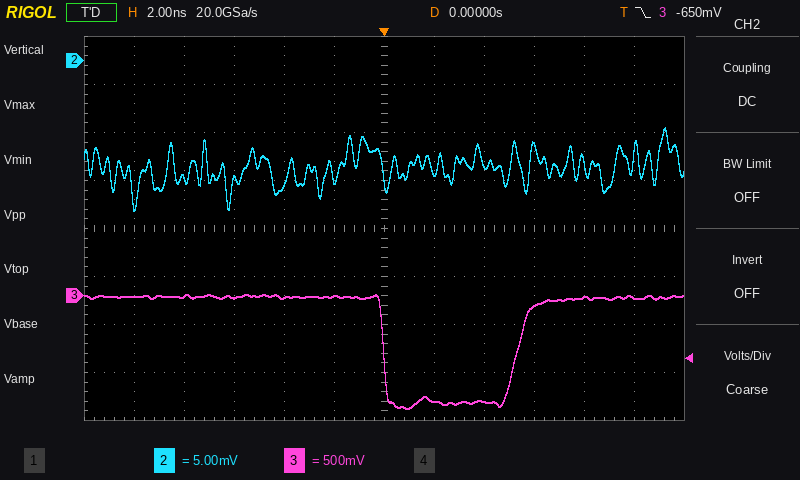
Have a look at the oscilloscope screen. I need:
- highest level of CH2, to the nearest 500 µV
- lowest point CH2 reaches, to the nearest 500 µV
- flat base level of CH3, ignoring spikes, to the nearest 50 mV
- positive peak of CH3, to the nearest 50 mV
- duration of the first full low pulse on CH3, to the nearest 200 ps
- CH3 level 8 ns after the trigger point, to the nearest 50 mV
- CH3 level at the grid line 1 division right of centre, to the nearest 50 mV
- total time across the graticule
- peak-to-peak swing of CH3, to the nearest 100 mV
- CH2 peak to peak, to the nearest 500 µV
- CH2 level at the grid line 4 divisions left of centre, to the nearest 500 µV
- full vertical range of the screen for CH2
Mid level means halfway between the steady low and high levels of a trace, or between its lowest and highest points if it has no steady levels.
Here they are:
-7.0 mV
-15.5 mV
-1.10 V
0 mV
5.4 ns
0 mV
-1.10 V
24 ns
1.20 V
8.5 mV
-12.5 mV
40 mV
